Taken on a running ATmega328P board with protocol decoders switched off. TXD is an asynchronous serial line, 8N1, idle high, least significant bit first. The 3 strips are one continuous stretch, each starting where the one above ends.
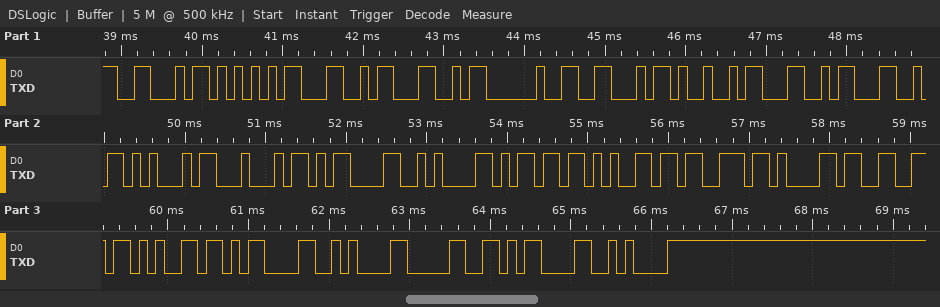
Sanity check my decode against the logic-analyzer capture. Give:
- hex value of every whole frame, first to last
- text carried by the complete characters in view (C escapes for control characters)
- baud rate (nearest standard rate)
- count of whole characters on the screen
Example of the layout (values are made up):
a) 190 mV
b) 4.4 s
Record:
a) 46 55 4C 4C 20 46 49 4C 4C 45 44 0D 0A 6D 65 73 61 66 65 0D 0A 30 0D 0A
b) "FULL FILLED\r\nmesafe\r\n0\r\n"
c) 9600 baud
d) 24
